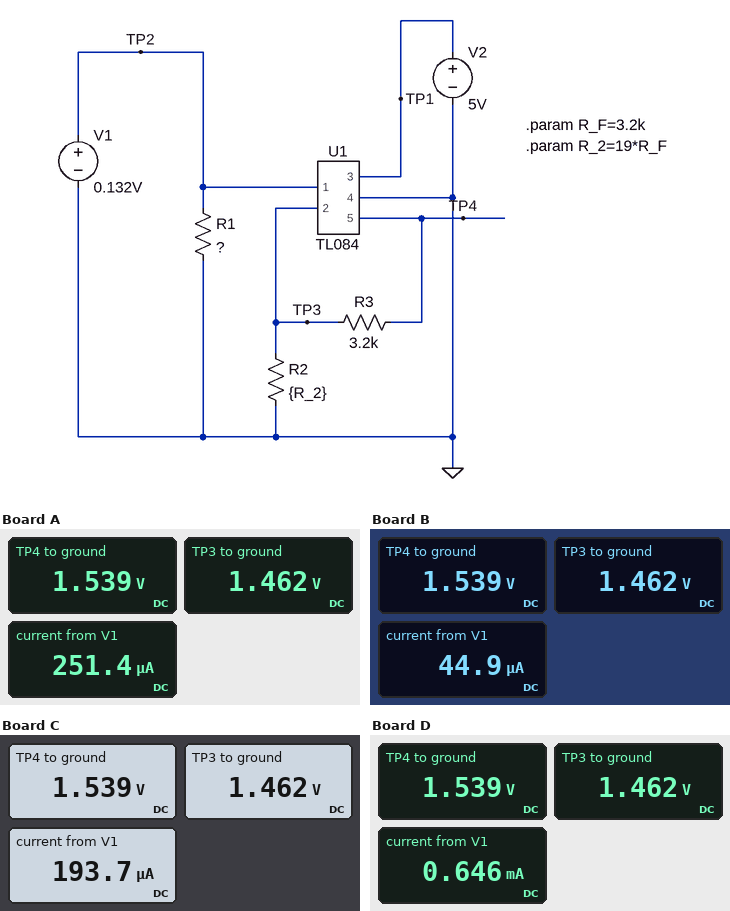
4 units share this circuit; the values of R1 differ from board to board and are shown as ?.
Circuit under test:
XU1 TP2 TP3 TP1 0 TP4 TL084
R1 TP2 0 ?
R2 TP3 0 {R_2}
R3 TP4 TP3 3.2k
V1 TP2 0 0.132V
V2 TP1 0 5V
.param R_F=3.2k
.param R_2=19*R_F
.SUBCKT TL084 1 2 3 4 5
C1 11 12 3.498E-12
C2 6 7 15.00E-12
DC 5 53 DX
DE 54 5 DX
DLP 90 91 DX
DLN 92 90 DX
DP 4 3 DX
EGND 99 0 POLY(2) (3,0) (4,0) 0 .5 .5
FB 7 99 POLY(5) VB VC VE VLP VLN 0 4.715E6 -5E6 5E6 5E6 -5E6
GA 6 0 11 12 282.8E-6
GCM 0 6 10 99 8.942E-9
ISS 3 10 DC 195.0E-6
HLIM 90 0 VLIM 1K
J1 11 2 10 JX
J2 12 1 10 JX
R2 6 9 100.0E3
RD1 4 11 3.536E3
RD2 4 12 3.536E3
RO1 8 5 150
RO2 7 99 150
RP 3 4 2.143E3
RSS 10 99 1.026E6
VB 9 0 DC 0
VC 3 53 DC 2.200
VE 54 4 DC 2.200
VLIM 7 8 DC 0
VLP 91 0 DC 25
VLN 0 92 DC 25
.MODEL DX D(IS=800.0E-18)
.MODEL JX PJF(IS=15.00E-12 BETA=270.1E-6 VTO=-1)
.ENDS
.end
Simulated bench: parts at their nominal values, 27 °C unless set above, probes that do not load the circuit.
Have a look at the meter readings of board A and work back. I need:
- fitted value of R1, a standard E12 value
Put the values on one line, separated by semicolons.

390 Ω
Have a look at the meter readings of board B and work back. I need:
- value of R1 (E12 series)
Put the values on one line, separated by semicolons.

1 kΩ
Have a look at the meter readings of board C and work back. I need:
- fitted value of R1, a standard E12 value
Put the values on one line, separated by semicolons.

470 Ω
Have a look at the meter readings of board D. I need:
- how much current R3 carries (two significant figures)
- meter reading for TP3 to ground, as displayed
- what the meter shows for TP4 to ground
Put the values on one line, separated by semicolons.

24 µA; 1.462 V; 1.539 V
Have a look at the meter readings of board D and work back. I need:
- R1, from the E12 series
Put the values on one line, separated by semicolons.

180 Ω
